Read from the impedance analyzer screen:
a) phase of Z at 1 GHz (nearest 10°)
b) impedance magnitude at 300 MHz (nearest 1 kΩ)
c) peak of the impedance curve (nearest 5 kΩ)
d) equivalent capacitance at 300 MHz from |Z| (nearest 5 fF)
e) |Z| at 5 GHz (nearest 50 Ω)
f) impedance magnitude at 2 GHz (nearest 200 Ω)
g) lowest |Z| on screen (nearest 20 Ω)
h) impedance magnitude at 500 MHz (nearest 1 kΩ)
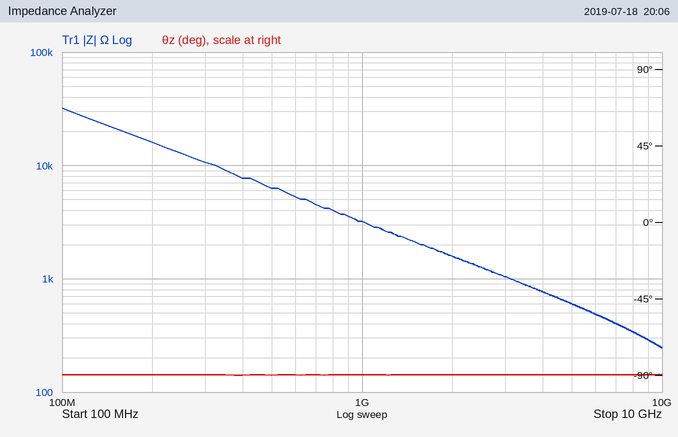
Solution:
-90°
11 kΩ
30 kΩ
50 fF
600 Ω
1.6 kΩ
240 Ω
6 kΩ
